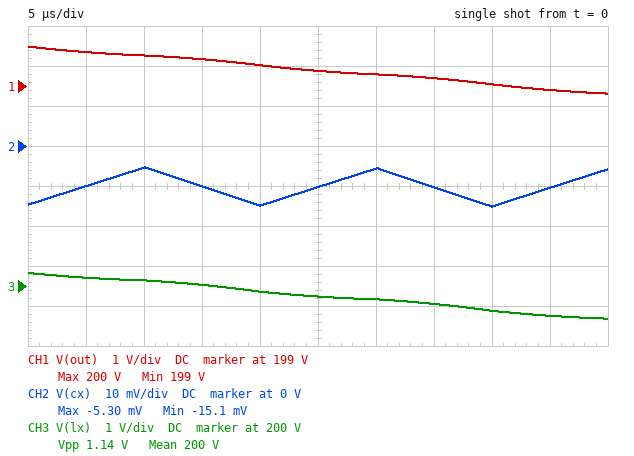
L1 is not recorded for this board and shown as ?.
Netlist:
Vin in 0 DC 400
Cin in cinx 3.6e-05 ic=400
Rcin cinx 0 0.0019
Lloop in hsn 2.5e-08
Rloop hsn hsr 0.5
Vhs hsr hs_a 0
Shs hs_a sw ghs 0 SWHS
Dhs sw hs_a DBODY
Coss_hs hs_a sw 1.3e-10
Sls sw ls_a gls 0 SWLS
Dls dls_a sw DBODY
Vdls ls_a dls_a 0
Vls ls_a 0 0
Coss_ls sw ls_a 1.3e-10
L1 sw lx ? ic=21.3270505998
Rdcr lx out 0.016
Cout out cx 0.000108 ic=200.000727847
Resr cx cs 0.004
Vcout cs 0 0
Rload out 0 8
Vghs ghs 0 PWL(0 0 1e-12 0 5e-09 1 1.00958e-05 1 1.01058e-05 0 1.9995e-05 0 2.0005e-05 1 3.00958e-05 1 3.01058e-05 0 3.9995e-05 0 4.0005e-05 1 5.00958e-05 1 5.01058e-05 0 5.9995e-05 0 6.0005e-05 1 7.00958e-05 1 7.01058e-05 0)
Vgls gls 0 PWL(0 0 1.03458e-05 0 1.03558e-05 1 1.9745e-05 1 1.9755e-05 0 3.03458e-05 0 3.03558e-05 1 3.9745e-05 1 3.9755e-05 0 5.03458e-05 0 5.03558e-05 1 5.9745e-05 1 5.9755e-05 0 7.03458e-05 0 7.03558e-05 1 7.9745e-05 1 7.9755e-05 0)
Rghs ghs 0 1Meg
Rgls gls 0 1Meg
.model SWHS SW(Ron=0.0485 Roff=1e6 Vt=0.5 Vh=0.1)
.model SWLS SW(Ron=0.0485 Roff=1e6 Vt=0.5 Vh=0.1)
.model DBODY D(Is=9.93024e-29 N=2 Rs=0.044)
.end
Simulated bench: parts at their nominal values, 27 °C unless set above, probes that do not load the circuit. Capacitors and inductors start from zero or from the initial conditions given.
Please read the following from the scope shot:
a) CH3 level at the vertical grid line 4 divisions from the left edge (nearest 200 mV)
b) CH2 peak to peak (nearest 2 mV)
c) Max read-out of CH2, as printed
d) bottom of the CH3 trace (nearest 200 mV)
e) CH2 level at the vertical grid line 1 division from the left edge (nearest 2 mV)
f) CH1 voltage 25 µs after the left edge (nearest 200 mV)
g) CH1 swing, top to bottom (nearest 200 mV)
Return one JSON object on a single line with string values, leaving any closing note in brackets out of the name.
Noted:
{"CH3 level at the vertical grid line 4 divisions from the left edge": "199.8 V", "CH2 peak to peak": "10 mV", "Max read-out of CH2, as printed": "-5.30 mV", "bottom of the CH3 trace": "199.2 V", "CH2 level at the vertical grid line 1 division from the left edge": "-10 mV", "CH1 voltage 25 µs after the left edge": "199.4 V", "CH1 swing, top to bottom": "1.2 V"}
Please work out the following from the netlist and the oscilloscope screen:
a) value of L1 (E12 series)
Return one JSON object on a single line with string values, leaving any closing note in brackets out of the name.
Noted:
{"value of L1": "820 µH"}
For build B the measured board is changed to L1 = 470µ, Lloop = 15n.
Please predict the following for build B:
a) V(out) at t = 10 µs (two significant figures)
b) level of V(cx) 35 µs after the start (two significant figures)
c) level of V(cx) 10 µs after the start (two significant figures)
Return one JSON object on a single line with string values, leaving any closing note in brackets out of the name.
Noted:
{"V(out) at t = 10 µs": "200 V", "level of V(cx) 35 µs after the start": "-7.6 mV", "level of V(cx) 10 µs after the start": "1.3 mV"}
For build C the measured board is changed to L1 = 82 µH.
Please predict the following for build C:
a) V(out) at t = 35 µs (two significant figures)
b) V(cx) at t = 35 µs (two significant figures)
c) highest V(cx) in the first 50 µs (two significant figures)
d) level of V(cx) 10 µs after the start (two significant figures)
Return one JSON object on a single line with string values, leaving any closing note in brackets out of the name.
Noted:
{"V(out) at t = 35 µs": "200 V", "V(cx) at t = 35 µs": "16 mV", "highest V(cx) in the first 50 µs": "74 mV", "level of V(cx) 10 µs after the start": "73 mV"}
